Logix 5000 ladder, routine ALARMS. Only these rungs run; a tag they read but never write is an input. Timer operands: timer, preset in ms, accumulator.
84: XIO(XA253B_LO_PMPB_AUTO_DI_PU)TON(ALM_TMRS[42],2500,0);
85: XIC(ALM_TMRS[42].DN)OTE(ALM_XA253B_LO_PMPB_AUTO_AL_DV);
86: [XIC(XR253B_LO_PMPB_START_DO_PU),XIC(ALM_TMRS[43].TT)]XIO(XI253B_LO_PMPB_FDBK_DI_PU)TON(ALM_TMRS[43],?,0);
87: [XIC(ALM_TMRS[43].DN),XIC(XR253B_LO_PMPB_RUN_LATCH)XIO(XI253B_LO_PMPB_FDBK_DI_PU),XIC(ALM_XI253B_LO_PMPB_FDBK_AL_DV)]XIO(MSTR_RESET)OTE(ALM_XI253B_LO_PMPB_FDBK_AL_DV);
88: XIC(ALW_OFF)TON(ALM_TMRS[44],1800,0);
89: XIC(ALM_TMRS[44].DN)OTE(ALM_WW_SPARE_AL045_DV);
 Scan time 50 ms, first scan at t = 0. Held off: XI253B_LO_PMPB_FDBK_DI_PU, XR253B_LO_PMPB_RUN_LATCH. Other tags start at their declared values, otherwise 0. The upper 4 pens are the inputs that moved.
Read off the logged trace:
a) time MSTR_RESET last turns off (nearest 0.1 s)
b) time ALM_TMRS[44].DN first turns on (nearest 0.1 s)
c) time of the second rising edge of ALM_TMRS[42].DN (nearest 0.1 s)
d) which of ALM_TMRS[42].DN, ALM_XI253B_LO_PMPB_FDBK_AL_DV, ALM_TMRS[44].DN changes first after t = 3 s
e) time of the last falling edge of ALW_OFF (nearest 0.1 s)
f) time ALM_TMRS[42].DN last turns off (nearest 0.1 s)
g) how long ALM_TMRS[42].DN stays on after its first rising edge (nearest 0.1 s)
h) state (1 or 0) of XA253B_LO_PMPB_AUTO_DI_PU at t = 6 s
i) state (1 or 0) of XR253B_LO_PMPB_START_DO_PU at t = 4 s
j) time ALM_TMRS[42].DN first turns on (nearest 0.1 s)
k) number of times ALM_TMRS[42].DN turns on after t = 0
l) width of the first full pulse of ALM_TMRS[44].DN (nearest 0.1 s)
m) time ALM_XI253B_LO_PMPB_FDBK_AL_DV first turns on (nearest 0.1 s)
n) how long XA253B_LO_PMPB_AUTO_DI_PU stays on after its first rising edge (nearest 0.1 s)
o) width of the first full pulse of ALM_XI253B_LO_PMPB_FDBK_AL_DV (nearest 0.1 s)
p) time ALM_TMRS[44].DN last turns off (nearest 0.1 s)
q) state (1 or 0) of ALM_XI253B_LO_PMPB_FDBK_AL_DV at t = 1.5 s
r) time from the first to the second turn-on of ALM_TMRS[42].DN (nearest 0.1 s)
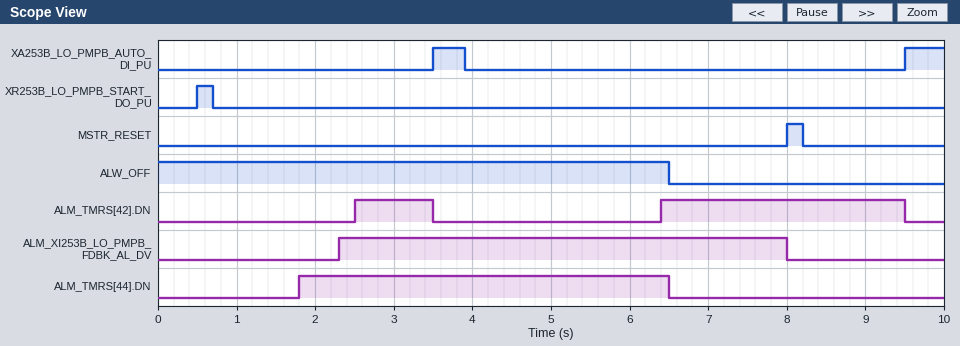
8.2 s
1.8 s
6.4 s
ALM_TMRS[42].DN
6.5 s
9.5 s
1.0 s
0
0
2.5 s
2
4.7 s
2.3 s
0.4 s
5.7 s
6.5 s
0
3.9 s
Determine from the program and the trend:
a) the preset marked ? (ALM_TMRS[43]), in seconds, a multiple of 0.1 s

1.8 s
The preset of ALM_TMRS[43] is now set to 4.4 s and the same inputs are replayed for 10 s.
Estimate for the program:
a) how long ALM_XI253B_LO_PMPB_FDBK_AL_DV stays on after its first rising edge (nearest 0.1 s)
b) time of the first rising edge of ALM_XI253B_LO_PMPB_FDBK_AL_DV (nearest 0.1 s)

3.1 s
4.9 s
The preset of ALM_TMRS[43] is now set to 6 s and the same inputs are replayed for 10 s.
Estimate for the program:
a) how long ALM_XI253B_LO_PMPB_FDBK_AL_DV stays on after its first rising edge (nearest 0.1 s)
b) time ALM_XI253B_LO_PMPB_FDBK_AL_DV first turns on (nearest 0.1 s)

1.5 s
6.5 s
